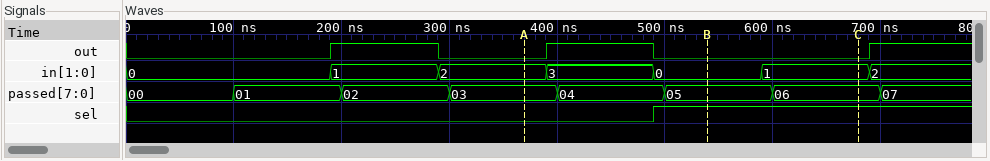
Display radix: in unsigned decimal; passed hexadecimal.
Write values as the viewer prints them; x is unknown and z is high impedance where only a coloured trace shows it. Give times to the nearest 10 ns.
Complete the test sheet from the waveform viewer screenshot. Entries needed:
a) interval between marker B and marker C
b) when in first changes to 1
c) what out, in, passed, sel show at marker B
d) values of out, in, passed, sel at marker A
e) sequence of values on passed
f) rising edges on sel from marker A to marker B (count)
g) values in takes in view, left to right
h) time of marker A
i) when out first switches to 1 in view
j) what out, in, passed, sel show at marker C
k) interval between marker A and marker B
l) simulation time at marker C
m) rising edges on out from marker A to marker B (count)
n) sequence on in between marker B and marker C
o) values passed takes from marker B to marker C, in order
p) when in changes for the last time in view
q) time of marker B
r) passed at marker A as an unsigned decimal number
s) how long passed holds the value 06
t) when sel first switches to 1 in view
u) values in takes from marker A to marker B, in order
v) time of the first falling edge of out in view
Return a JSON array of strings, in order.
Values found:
["140 ns", "190 ns", "out=0, in=0, passed=05, sel=1", "out=0, in=2, passed=03, sel=0", "00, 01, 02, 03, 04, 05, 06, 07", "1", "0, 1, 2, 3, 0, 1, 2", "370 ns", "190 ns", "out=0, in=1, passed=06, sel=1", "170 ns", "680 ns", "1", "0, 1", "05, 06", "690 ns", "540 ns", "3", "100 ns", "490 ns", "2, 3, 0", "290 ns"]
